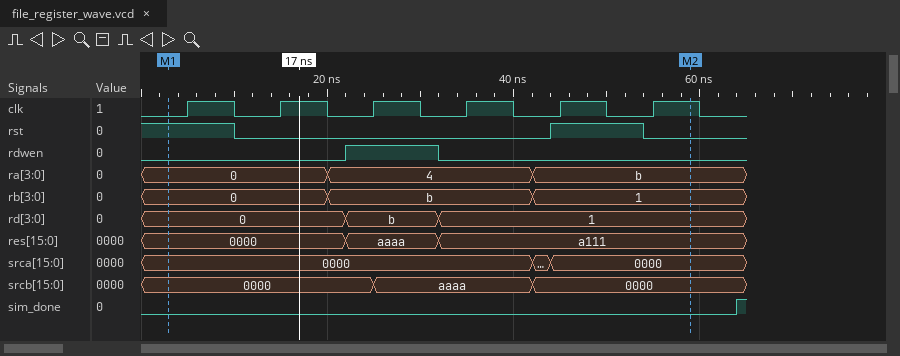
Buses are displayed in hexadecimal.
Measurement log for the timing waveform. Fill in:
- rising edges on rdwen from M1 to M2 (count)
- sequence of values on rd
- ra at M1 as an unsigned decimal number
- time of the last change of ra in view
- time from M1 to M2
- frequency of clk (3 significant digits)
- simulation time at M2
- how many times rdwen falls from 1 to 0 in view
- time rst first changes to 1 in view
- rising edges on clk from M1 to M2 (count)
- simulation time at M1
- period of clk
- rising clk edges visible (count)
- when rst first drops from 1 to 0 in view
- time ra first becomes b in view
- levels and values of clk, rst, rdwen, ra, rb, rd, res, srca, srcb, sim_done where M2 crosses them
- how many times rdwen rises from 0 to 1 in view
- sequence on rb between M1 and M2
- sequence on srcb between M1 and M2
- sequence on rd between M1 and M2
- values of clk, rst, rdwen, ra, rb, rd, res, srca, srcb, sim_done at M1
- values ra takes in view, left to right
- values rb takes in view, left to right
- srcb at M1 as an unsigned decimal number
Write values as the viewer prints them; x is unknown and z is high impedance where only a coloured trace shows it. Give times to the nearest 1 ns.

1
0, b, 1
0
42 ns
56 ns
100 MHz
59 ns
1
44 ns
6
3 ns
10 ns
6
10 ns
42 ns
clk=1, rst=0, rdwen=0, ra=b, rb=1, rd=1, res=a111, srca=0000, srcb=0000, sim_done=0
1
0, b, 1
0000, aaaa, 0000
0, b, 1
clk=0, rst=1, rdwen=0, ra=0, rb=0, rd=0, res=0000, srca=0000, srcb=0000, sim_done=0
0, 4, b
0, b, 1
0
